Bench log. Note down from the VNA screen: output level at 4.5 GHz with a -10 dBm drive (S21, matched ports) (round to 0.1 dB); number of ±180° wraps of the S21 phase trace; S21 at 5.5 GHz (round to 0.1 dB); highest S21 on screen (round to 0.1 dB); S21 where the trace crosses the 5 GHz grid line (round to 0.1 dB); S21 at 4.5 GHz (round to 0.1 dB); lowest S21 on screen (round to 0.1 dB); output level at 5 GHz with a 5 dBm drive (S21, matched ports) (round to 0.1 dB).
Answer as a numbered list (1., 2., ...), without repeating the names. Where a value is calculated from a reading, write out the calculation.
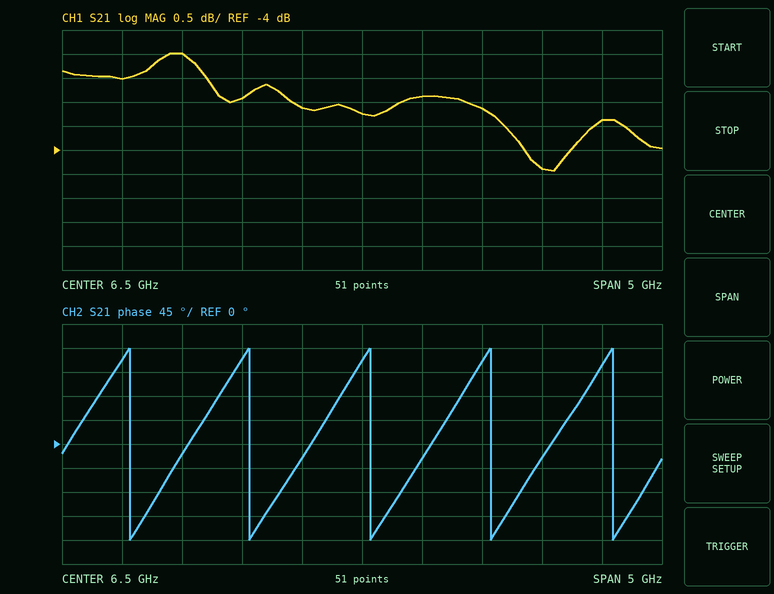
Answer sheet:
1. -10 dBm + (-2.5 dB) = -12.5 dBm
2. 5
3. -2.9 dB
4. -2.0 dB
5. -2.0 dB
6. -2.5 dB
7. -4.4 dB
8. 5 dBm + (-2.0 dB) = 3.0 dBm
